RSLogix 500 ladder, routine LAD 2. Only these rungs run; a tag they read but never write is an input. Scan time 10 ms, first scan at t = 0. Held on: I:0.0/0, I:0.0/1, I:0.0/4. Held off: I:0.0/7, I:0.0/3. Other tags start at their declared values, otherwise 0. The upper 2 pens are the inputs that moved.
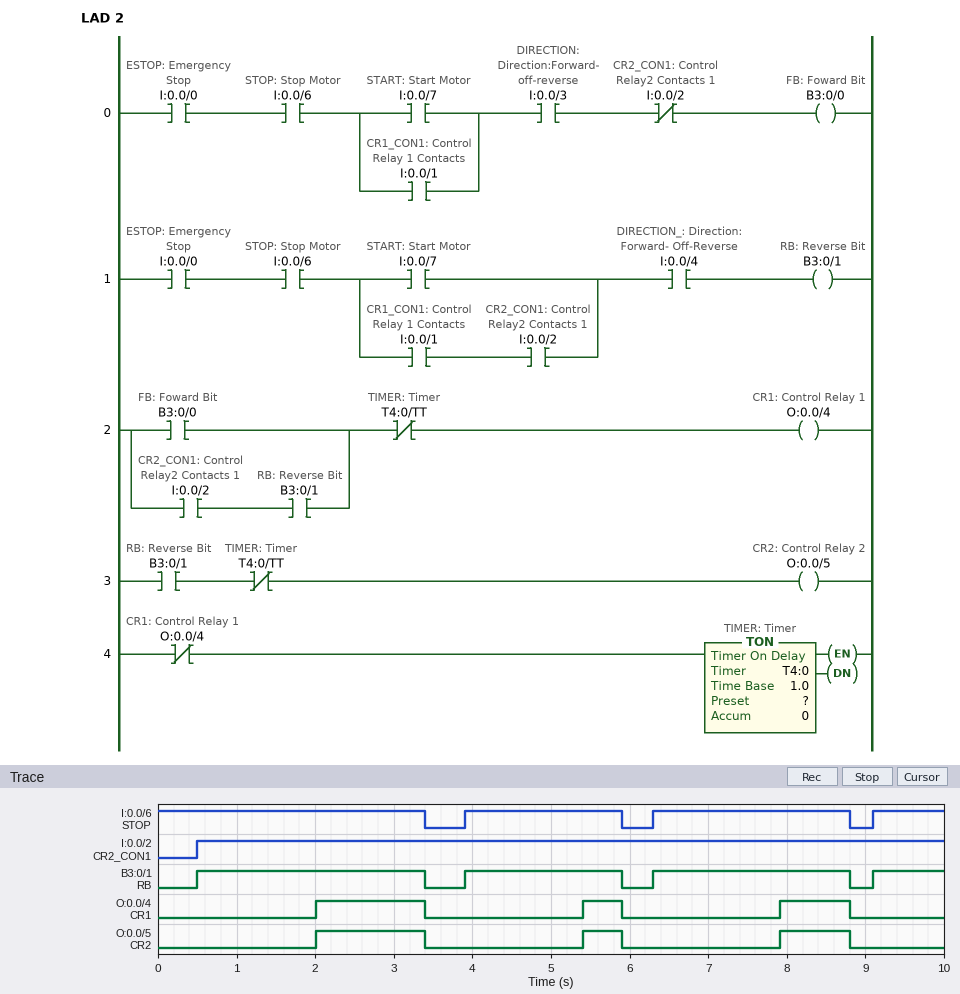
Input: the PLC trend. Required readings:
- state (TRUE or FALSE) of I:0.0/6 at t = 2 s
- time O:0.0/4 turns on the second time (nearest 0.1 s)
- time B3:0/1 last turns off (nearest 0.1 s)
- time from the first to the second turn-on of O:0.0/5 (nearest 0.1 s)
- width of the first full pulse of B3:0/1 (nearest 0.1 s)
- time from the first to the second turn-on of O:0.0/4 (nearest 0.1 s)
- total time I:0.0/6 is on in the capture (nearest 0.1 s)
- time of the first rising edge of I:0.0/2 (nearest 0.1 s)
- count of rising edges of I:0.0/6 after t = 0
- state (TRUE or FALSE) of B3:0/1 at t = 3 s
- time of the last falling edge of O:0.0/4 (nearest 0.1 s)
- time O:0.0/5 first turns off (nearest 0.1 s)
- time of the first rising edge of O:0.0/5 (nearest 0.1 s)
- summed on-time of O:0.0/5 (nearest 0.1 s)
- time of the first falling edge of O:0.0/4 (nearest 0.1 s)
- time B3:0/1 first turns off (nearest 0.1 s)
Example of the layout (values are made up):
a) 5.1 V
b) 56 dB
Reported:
a) TRUE
b) 5.4 s
c) 8.8 s
d) 3.4 s
e) 2.9 s
f) 3.4 s
g) 8.8 s
h) 0.5 s
i) 3
j) TRUE
k) 8.8 s
l) 3.4 s
m) 2.0 s
n) 2.8 s
o) 3.4 s
p) 3.4 s
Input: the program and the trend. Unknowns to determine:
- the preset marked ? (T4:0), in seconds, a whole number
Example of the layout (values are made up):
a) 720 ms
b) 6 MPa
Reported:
a) 2 s
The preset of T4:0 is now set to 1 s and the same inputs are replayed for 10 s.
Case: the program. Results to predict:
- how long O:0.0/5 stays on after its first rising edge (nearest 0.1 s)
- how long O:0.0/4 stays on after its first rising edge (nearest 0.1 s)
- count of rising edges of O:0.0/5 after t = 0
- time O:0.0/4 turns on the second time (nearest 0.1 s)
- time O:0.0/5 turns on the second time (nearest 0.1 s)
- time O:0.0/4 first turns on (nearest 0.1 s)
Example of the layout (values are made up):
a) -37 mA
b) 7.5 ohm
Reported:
a) 2.4 s
b) 2.4 s
c) 4
d) 4.4 s
e) 4.4 s
f) 1.0 s
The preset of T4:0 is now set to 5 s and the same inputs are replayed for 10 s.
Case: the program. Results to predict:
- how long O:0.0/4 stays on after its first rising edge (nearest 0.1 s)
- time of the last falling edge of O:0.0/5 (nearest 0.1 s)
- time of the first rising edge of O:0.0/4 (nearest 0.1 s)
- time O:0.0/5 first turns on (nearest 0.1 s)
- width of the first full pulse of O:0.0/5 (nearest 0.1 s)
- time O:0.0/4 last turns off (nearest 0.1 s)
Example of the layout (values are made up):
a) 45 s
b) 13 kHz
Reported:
a) 0.9 s
b) 5.9 s
c) 5.0 s
d) 5.0 s
e) 0.9 s
f) 5.9 s
